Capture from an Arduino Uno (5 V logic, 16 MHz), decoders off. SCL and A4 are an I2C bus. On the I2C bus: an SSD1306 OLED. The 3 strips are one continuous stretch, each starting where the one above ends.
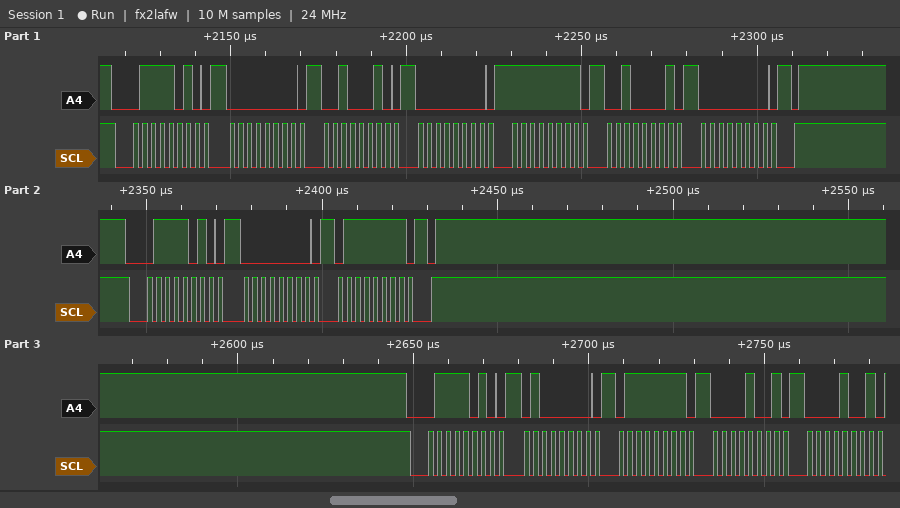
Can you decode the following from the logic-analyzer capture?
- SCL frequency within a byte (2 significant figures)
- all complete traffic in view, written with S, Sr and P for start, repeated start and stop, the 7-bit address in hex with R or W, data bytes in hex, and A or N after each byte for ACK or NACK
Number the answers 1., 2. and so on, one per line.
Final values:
1. 400 kHz
2. S 3DW A 00 A 22 A 00 A FF A 21 A 00 A P S 3DW A 00 A 7F A P S 3DW A 40 A 7F A 09 A 09 A
